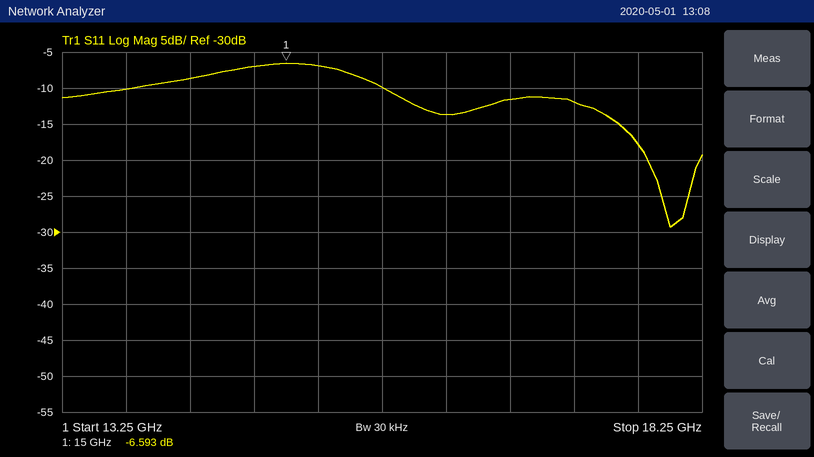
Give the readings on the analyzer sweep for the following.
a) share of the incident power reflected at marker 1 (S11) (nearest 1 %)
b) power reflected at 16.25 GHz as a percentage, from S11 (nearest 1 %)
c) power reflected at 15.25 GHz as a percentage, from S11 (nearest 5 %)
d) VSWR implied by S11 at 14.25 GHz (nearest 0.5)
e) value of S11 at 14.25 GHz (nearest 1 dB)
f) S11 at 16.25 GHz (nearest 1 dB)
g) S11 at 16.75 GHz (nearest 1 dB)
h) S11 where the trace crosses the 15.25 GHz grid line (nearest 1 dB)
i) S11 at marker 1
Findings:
22 %
4 %
20 %
2.0
-9 dB
-14 dB
-12 dB
-7 dB
-6.593 dB
